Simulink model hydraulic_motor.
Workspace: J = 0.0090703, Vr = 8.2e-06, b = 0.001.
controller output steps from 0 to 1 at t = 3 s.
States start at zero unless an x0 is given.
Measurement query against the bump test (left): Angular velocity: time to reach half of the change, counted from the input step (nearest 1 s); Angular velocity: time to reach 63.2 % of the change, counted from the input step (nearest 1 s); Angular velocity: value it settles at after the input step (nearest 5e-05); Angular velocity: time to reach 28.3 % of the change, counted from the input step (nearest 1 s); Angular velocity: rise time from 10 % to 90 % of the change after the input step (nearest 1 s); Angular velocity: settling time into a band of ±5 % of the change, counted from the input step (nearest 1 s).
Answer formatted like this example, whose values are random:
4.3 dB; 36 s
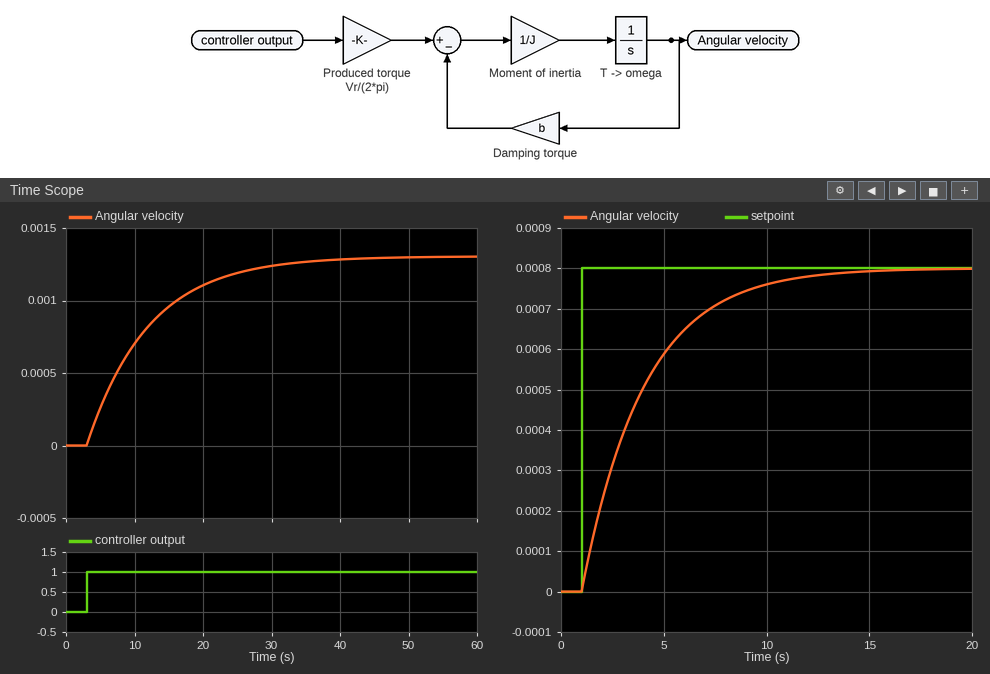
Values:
6 s; 9 s; 0.00130; 3 s; 20 s; 27 s
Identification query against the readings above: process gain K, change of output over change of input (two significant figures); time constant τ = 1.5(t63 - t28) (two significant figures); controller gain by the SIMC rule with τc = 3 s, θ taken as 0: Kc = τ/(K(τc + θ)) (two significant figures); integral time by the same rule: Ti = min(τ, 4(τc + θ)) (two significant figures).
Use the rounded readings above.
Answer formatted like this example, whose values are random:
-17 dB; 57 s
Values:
0.0013; 9.0 s; 2300; 9.0 s
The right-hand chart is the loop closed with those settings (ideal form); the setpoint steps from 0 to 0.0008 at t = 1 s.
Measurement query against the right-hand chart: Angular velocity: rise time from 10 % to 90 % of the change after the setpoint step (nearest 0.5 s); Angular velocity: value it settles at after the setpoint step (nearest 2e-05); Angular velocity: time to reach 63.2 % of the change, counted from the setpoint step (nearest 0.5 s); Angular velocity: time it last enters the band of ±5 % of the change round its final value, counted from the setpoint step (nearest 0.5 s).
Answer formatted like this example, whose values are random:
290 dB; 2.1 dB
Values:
6.5 s; 0.00080; 3.0 s; 9.0 s
